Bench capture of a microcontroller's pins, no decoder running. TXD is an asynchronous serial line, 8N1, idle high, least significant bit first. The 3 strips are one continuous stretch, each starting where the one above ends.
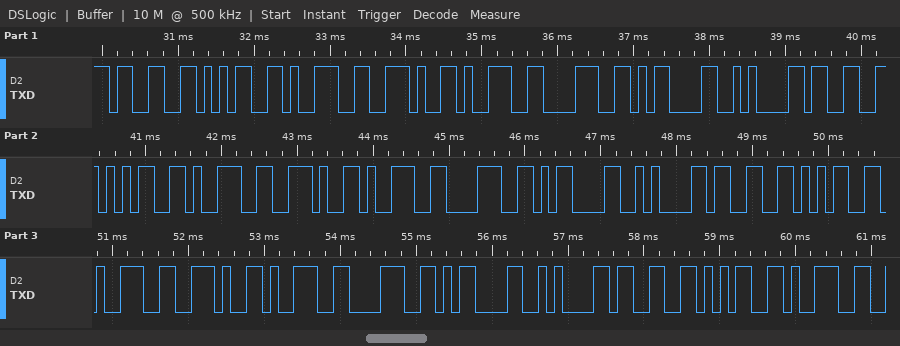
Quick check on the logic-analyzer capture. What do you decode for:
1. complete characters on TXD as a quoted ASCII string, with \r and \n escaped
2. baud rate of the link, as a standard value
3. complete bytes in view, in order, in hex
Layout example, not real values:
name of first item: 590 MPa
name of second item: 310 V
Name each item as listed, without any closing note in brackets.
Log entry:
complete characters on TXD as a quoted ASCII string, with \r and \n escaped: "359.98\r\n359.98\r\n359.98\r\n359"
baud rate of the link, as a standard value: 9600 baud
complete bytes in view, in order, in hex: 33 35 39 2E 39 38 0D 0A 33 35 39 2E 39 38 0D 0A 33 35 39 2E 39 38 0D 0A 33 35 39
